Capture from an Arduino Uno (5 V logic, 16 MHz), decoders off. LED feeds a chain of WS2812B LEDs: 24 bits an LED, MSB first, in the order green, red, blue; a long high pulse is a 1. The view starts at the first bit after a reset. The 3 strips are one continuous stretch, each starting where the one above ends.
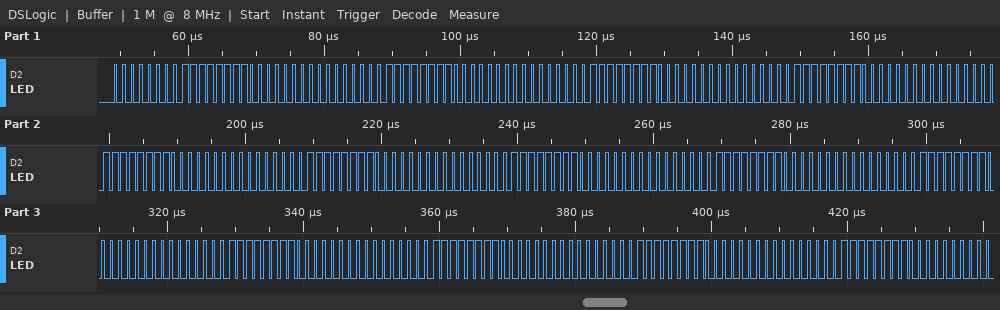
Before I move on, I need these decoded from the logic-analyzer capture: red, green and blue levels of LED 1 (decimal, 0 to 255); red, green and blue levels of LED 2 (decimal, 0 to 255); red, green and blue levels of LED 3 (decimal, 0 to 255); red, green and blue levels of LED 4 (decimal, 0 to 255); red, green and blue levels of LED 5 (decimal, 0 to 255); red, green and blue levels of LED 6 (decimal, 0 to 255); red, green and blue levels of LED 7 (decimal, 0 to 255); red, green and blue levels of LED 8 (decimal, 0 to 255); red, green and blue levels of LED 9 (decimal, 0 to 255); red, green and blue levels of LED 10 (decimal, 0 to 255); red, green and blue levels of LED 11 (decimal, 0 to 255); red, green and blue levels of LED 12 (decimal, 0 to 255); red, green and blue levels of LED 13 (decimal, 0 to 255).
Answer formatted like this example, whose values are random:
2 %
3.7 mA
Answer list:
255, 0, 0
255, 0, 0
255, 0, 0
255, 0, 0
255, 0, 0
255, 0, 0
255, 0, 0
255, 0, 0
255, 0, 0
255, 0, 0
255, 0, 0
255, 0, 0
255, 0, 0
